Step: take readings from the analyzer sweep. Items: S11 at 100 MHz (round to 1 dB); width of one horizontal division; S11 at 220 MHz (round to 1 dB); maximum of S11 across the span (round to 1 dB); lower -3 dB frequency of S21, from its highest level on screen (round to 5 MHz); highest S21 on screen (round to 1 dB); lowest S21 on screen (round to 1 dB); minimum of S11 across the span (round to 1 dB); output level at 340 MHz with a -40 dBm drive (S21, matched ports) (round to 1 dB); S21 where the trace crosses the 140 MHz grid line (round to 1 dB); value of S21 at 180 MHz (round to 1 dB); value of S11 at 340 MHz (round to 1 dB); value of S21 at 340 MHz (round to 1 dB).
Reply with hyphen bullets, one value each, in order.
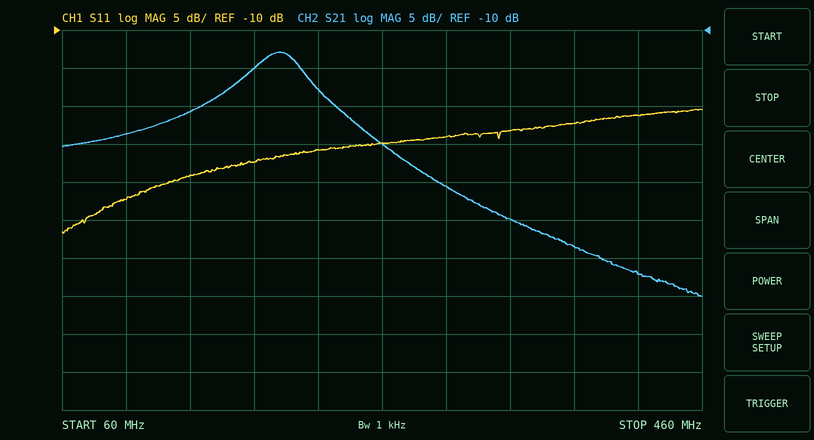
- -32 dB
- 40 MHz
- -26 dB
- -20 dB
- 175 MHz
- -13 dB
- -45 dB
- -37 dB
- -75 dBm
- -21 dB
- -15 dB
- -23 dB
- -35 dB
